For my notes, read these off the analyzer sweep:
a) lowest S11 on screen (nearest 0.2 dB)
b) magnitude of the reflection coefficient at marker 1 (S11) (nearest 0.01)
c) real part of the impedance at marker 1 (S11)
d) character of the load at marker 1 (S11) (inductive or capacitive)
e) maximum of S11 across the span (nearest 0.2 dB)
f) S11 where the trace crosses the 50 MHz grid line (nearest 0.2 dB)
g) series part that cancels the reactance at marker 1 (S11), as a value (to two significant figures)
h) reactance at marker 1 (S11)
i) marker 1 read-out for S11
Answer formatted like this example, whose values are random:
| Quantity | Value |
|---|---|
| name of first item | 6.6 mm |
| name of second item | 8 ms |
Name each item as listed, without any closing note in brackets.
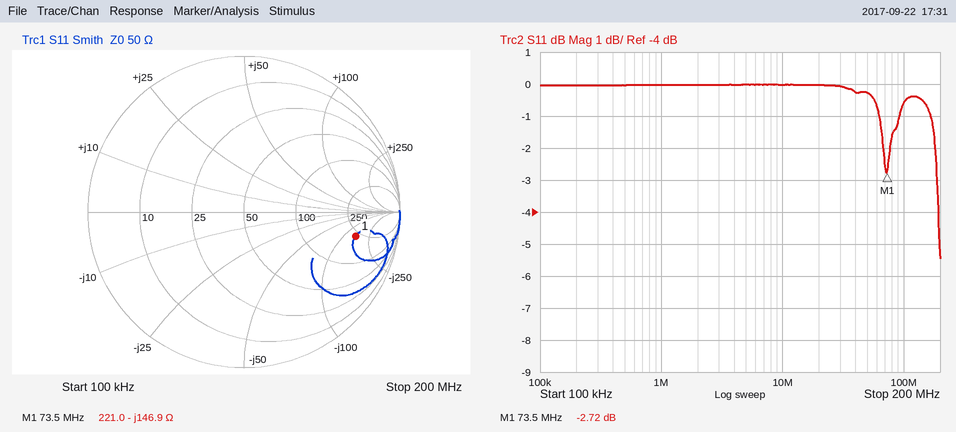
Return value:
| Quantity | Value |
|---|---|
| lowest S11 on screen | -5.4 dB |
| magnitude of the reflection coefficient at marker 1 (S11) | 0.73 |
| real part of the impedance at marker 1 | 221.0 Ω |
| character of the load at marker 1 (S11) | capacitive |
| maximum of S11 across the span | 0.0 dB |
| S11 where the trace crosses the 50 MHz grid line | -0.2 dB |
| series part that cancels the reactance at marker 1 (S11), as a value | 320 nH |
| reactance at marker 1 | -146.9 Ω |
| marker 1 read-out for S11 | -2.72 dB |
